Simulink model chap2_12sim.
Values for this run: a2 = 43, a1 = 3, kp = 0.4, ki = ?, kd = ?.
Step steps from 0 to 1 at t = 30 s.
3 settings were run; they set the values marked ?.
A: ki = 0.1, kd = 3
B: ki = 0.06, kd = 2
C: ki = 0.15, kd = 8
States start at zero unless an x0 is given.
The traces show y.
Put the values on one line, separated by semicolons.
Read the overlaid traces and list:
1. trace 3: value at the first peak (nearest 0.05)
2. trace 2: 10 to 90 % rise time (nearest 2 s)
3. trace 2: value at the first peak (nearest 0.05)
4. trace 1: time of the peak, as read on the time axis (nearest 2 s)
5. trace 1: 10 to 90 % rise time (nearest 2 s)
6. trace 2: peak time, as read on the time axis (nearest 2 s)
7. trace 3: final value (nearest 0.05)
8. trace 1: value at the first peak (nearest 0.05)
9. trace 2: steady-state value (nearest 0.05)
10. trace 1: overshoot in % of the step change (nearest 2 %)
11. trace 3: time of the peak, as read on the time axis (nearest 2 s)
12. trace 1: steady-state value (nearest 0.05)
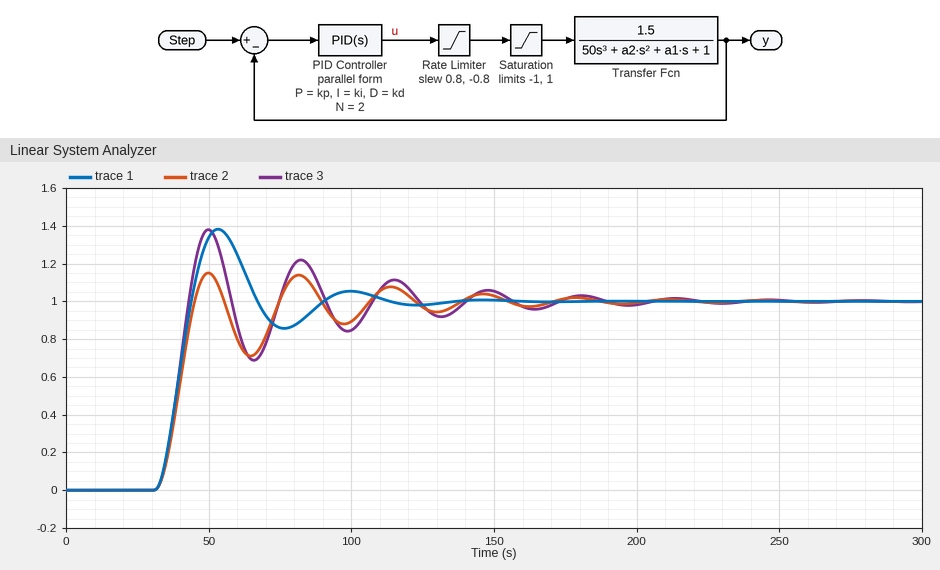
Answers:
1.40; 10 s; 1.15; 54 s; 8 s; 50 s; 1.00; 1.40; 1.00; 38 %; 50 s; 1.00
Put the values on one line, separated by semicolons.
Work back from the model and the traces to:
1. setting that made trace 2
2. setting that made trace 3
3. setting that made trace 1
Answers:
B; A; C
